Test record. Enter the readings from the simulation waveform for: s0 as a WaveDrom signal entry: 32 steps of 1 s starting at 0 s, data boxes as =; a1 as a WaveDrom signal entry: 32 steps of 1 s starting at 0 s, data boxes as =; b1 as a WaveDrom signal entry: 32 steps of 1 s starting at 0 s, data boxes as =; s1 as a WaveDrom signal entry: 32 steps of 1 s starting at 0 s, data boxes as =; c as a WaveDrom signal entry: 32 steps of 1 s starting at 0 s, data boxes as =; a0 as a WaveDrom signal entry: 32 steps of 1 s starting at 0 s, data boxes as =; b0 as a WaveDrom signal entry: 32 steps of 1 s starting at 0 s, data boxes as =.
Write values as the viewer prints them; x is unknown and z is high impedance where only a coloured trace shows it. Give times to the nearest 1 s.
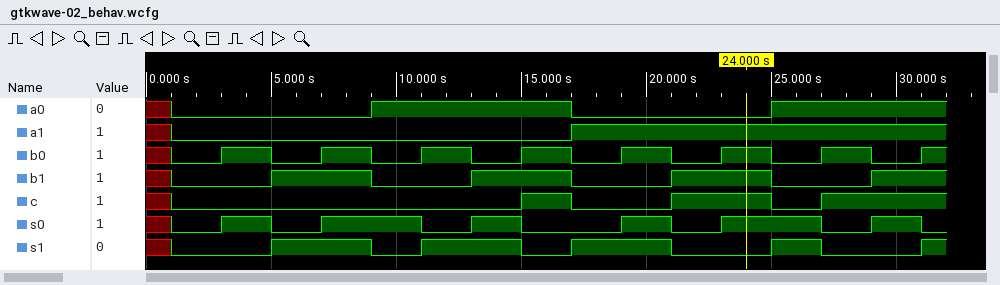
{name: 's0', wave: 'x0.1.0.1...0.1.0...1.0.1...0.1.0'}
{name: 'a1', wave: 'x0...............1..............'}
{name: 'b1', wave: 'x0...1...0...1...0...1...0...1..'}
{name: 's1', wave: 'x0...1...0.1...0.1...0...1.0...1'}
{name: 'c', wave: 'x0.............1.0...1...0.1....'}
{name: 'a0', wave: 'x0.......1.......0.......1......'}
{name: 'b0', wave: 'x0.1.0.1.0.1.0.1.0.1.0.1.0.1.0.1'}
